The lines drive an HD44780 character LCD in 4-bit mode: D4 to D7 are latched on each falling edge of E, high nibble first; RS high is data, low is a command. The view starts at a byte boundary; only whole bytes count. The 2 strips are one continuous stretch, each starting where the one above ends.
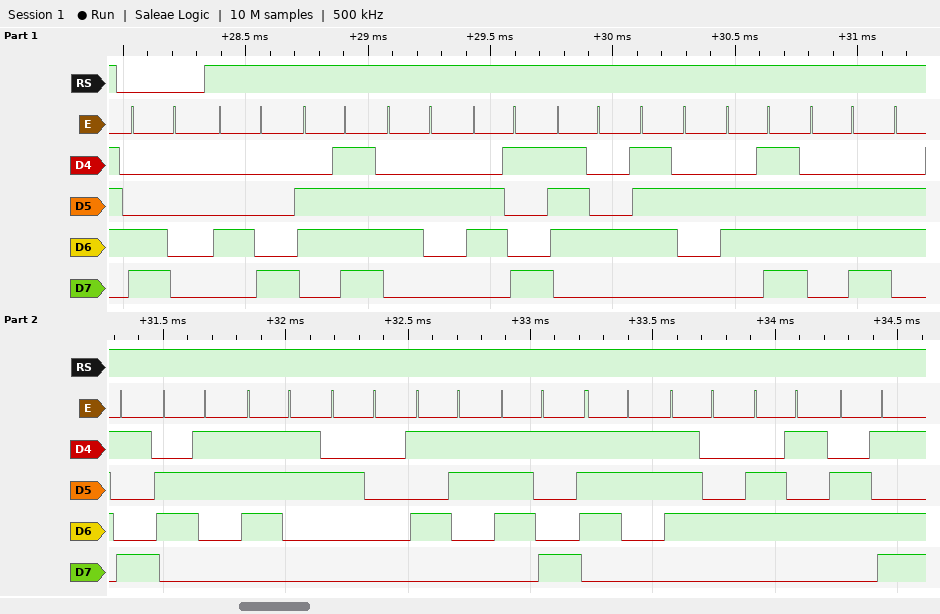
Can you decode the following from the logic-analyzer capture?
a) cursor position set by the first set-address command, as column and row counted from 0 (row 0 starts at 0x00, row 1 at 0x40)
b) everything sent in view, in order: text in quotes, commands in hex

column 0, row 1
0xC0 "Hobitronics System"
